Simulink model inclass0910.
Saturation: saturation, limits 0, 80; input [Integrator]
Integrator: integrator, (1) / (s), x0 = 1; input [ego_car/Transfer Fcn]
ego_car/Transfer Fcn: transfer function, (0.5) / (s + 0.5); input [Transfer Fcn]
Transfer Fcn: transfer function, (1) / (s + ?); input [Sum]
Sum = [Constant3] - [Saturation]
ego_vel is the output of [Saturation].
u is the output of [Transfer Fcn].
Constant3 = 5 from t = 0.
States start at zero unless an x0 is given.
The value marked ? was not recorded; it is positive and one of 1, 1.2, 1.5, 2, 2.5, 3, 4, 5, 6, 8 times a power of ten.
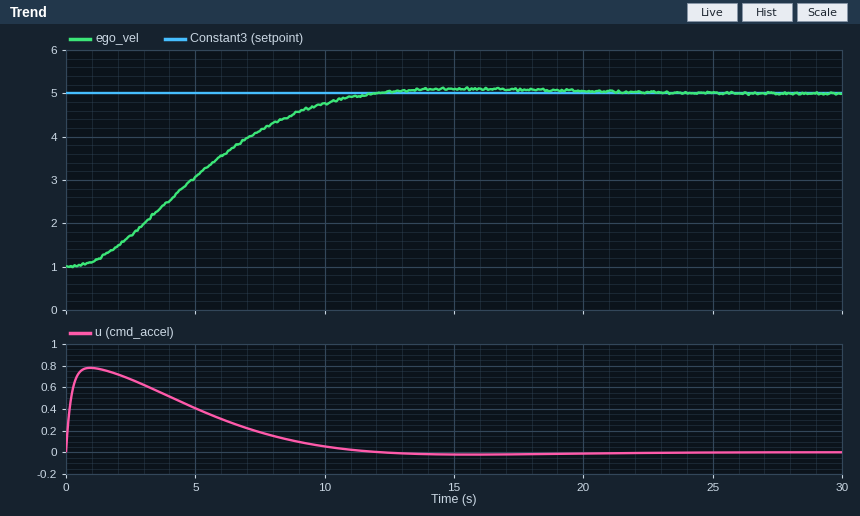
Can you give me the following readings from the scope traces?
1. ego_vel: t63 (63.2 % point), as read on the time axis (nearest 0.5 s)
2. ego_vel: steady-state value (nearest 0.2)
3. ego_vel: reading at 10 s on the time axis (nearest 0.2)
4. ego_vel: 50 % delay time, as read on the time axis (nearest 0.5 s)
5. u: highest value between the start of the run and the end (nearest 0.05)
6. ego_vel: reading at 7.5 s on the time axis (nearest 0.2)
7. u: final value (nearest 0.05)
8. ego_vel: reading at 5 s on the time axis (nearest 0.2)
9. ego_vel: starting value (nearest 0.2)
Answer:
6.0 s
5.0
4.8
5.0 s
0.80
4.2
0.00
3.0
1.0
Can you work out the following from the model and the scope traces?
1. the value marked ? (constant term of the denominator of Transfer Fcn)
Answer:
5
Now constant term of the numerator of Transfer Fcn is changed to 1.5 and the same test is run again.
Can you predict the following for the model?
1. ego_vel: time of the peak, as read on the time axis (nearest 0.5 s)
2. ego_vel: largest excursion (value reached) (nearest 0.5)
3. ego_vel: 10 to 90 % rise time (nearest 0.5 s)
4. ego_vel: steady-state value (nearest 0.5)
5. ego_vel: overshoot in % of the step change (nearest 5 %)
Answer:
10.5 s
5.5
5.0 s
5.0
10 %
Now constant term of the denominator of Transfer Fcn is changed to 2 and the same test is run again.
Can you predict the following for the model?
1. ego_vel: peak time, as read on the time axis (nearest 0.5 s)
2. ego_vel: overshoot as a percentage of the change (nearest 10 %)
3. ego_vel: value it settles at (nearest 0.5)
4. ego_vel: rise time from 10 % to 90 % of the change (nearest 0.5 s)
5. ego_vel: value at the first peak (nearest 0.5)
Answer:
7.5 s
30 %
5.0
3.0 s
6.0
